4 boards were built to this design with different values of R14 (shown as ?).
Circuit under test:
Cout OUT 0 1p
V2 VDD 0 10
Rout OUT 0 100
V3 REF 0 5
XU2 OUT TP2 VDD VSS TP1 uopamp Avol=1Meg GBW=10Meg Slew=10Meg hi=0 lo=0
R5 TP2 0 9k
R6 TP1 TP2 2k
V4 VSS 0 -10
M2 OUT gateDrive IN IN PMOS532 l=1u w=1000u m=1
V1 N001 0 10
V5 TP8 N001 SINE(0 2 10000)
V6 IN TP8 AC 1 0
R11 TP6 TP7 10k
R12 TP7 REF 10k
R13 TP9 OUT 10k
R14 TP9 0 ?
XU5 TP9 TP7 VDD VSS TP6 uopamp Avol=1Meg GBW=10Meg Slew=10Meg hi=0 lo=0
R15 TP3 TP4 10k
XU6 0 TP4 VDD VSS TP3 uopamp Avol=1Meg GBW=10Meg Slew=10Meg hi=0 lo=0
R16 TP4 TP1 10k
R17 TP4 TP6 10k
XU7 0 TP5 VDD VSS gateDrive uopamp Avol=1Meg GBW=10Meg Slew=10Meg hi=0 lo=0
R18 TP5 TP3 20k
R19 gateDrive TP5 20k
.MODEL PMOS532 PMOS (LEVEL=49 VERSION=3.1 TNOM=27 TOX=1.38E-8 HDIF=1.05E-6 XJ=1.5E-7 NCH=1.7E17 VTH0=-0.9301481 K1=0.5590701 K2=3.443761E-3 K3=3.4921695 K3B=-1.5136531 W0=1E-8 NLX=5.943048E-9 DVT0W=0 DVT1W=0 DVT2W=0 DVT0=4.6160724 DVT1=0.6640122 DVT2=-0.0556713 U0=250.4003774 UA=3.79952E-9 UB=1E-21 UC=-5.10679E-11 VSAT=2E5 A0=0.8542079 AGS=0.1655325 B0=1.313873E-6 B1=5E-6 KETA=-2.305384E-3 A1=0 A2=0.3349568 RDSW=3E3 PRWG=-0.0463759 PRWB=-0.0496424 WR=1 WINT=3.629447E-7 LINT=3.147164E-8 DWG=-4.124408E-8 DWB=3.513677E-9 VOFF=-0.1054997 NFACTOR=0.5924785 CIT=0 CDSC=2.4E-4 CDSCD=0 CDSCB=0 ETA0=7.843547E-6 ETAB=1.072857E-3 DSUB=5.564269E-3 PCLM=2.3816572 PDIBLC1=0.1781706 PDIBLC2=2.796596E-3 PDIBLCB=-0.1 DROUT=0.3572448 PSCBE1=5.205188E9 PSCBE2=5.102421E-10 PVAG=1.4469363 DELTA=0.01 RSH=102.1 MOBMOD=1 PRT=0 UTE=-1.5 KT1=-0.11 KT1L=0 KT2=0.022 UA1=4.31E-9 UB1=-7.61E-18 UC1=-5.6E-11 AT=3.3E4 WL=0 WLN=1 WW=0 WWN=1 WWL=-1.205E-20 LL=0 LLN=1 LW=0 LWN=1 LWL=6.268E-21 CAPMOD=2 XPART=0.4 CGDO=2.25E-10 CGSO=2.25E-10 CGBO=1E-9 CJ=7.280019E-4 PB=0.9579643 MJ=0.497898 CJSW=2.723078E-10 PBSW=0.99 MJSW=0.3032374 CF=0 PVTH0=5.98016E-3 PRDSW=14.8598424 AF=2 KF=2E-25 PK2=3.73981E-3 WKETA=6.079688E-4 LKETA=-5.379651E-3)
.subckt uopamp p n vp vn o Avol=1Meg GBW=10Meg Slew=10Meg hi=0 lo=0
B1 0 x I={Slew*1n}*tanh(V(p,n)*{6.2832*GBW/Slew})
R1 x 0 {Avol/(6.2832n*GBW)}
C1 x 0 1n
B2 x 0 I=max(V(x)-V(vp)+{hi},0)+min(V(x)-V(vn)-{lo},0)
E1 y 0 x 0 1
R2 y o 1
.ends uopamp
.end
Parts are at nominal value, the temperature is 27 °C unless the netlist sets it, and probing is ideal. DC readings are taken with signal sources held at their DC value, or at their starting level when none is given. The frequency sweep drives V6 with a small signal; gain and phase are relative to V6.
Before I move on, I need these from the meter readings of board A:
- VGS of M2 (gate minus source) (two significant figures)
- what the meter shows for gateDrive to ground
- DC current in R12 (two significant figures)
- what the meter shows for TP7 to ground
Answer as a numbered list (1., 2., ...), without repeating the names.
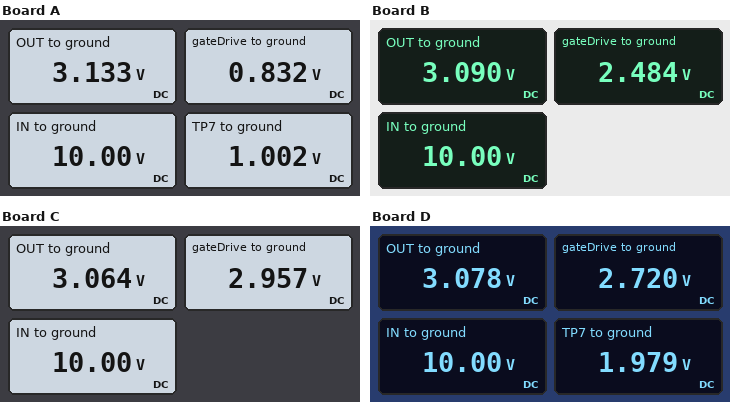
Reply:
1. -9.2 V
2. 0.832 V
3. 400 µA
4. 1.002 V
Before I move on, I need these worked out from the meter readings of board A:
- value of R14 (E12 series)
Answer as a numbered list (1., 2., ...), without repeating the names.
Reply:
1. 4.7 kΩ
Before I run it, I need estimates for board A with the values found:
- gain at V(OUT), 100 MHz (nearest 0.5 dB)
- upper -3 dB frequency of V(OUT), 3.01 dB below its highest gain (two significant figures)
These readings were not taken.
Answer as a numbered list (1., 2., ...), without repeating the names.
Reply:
1. -10.0 dB
2. 800 MHz
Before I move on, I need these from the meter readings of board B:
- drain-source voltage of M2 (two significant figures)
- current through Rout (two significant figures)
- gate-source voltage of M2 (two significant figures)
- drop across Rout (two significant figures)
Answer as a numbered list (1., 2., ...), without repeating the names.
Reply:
1. -6.9 V
2. 31 mA
3. -7.5 V
4. 3.1 V
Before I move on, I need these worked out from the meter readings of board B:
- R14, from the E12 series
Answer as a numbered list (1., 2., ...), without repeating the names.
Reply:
1. 15 kΩ
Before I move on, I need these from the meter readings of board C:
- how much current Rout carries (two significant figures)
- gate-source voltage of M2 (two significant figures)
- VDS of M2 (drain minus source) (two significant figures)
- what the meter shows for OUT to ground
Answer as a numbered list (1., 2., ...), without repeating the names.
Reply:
1. 31 mA
2. -7.0 V
3. -6.9 V
4. 3.064 V
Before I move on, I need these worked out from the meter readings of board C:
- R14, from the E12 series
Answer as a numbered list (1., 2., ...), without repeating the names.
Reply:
1. 22 kΩ
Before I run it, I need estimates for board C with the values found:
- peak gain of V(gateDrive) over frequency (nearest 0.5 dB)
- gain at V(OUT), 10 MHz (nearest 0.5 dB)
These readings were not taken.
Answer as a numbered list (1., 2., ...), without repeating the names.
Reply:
1. -2.5 dB
2. -9.0 dB
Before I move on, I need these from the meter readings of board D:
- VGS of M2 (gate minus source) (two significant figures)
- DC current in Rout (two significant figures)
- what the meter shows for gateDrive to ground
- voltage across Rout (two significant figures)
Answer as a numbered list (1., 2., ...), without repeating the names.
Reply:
1. -7.3 V
2. 31 mA
3. 2.720 V
4. 3.1 V
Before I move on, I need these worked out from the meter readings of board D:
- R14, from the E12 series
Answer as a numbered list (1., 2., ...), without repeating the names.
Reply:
1. 18 kΩ
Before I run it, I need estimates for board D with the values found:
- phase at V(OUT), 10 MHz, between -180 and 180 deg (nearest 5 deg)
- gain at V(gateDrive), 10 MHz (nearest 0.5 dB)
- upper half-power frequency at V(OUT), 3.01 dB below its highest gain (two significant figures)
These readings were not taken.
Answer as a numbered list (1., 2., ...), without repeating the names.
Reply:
1. 0 deg
2. -23.5 dB
3. 650 MHz
